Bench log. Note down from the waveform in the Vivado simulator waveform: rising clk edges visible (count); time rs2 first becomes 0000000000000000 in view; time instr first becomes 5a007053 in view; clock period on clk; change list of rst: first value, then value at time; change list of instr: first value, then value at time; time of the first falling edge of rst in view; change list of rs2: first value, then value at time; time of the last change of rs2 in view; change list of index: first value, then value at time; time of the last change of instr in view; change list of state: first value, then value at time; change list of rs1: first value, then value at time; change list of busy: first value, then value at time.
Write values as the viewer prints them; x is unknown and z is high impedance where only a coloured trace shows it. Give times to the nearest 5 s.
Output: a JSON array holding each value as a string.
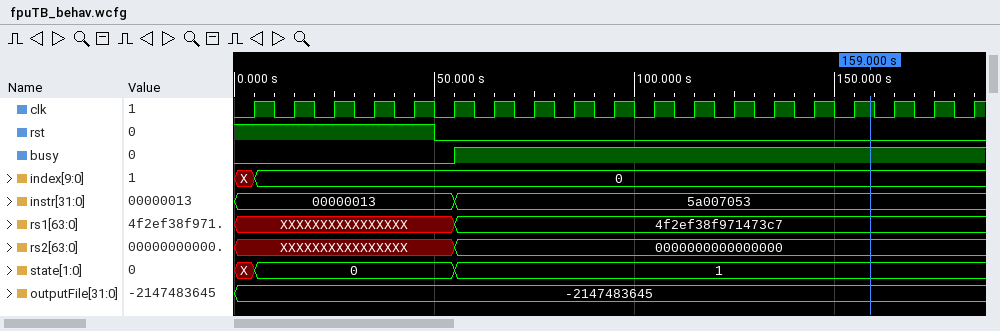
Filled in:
["19", "55 s", "55 s", "10 s", "1, 0 at 50 s", "00000013, 5a007053 at 55 s", "50 s", "XXXXXXXXXXXXXXXX, 0000000000000000 at 55 s", "55 s", "X, 0 at 5 s", "55 s", "X, 0 at 5 s, 1 at 55 s", "XXXXXXXXXXXXXXXX, 4f2ef38f971473c7 at 55 s", "0, 1 at 55 s"]
